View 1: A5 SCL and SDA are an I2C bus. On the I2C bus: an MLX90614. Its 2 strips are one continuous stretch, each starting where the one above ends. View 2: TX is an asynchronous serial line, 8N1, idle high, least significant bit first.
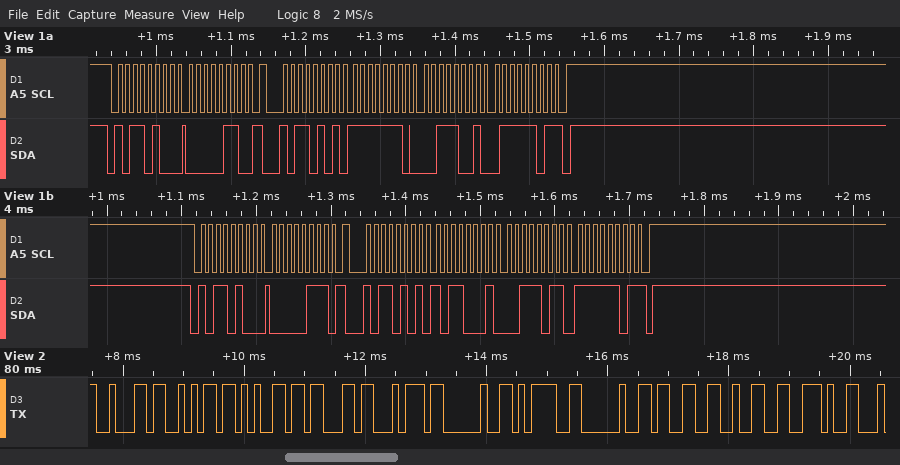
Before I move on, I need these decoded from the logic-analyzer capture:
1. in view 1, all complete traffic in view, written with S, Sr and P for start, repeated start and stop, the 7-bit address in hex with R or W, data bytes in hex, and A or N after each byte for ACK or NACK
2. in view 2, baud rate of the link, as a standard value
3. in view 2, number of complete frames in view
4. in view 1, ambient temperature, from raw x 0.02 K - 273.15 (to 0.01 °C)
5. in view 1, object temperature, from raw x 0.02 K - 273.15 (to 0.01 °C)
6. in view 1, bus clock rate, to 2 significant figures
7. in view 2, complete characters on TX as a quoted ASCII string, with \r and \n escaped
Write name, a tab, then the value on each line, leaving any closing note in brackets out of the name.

in view 1, all complete traffic in view, written with S, Sr and P for start, repeated start and stop, the 7-bit address in hex with R or W, data bytes in hex, and A or N after each byte for ACK or NACK	S 5AW A 06 A Sr 5AR A FE A 39 A 7D N P S 5AW A 07 A Sr 5AR A B1 A 3B A FD N P
in view 2, baud rate of the link, as a standard value	9600 baud
in view 2, number of complete frames in view	11
in view 1, ambient temperature, from raw x 0.02 K - 273.15	23.77 °C
in view 1, object temperature, from raw x 0.02 K - 273.15	32.47 °C
in view 1, bus clock rate, to 2 significant figures	100 kHz
in view 2, complete characters on TX as a quoted ASCII string, with \r and \n escaped	"bject = 32."
